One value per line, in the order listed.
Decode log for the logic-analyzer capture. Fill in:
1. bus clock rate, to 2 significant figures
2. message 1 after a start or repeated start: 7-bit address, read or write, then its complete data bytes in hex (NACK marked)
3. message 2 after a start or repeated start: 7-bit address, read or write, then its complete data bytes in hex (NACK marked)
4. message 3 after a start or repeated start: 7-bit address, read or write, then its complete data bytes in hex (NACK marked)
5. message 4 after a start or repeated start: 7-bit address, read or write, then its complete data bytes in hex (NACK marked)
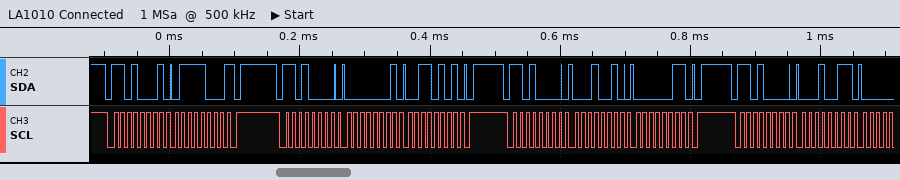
100 kHz
0x68 read: 78 NACK
0x68 write: 01 35
0x68 write: 12 03
0x68 write: 13
